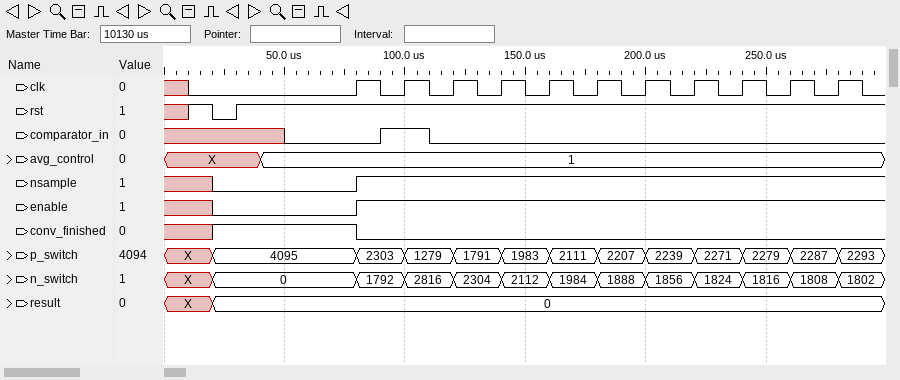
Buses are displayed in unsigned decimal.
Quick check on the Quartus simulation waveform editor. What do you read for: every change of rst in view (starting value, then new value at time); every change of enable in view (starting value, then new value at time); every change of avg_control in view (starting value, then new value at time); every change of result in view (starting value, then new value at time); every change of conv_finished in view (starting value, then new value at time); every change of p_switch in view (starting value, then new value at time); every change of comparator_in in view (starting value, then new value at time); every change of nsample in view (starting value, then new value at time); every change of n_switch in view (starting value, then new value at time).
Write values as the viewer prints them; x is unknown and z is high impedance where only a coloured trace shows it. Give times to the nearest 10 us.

x, 1 at 10 us, 0 at 20 us, 1 at 30 us
x, 0 at 20 us, 1 at 80 us
X, 1 at 40 us
X, 0 at 20 us
x, 1 at 20 us, 0 at 80 us
X, 4095 at 20 us, 2303 at 80 us, 1279 at 100 us, 1791 at 120 us, 1983 at 140 us, 2111 at 160 us, 2207 at 180 us, 2239 at 200 us, 2271 at 220 us, 2279 at 240 us, 2287 at 260 us, 2293 at 280 us
x, 0 at 50 us, 1 at 90 us, 0 at 110 us
x, 0 at 20 us, 1 at 80 us
X, 0 at 20 us, 1792 at 80 us, 2816 at 100 us, 2304 at 120 us, 2112 at 140 us, 1984 at 160 us, 1888 at 180 us, 1856 at 200 us, 1824 at 220 us, 1816 at 240 us, 1808 at 260 us, 1802 at 280 us
